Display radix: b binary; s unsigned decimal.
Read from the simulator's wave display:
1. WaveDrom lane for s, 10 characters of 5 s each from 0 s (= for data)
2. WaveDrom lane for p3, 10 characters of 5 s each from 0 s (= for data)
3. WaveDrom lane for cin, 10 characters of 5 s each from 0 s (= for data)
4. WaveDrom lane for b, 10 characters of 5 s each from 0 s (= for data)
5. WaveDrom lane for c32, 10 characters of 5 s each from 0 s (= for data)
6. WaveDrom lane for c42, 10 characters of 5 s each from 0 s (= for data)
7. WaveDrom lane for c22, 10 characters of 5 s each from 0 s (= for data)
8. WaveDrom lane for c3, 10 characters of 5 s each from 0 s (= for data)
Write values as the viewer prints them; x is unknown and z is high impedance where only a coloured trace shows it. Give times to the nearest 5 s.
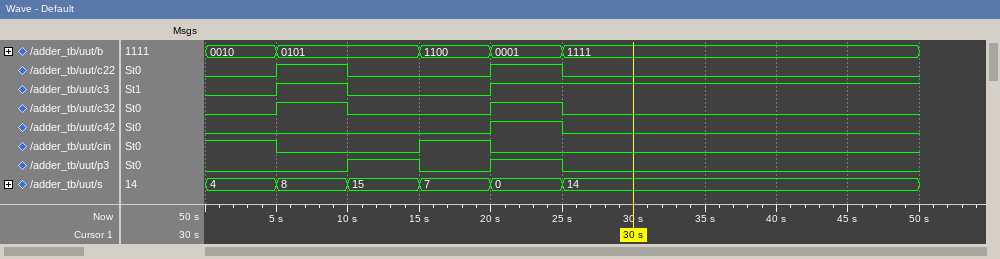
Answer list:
{name: 's', wave: '======....', data: '4 8 15 7 0 14'}
{name: 'p3', wave: '0.1010....'}
{name: 'cin', wave: '10.10.....'}
{name: 'b', wave: '==.===....', data: '0010 0101 1100 0001 1111'}
{name: 'c32', wave: '010.10....'}
{name: 'c42', wave: '0...10....'}
{name: 'c22', wave: '010.10....'}
{name: 'c3', wave: '010.1.....'}
